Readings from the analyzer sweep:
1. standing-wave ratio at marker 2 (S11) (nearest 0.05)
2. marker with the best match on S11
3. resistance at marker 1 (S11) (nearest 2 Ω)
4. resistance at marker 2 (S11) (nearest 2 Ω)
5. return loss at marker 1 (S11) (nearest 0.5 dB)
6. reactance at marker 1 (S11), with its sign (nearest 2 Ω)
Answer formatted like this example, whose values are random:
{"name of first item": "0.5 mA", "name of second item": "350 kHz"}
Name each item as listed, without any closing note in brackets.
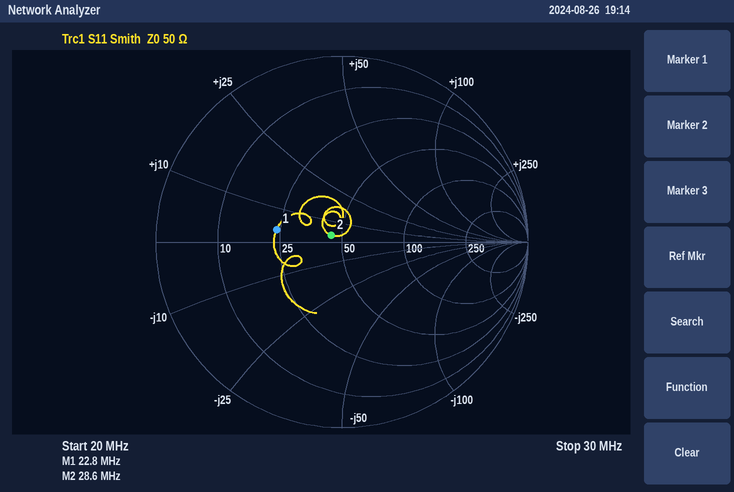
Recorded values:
{"standing-wave ratio at marker 2 (S11)": "1.15", "marker with the best match on S11": "marker 2", "resistance at marker 1 (S11)": "24 Ω", "resistance at marker 2 (S11)": "44 Ω", "return loss at marker 1 (S11)": "9.0 dB", "reactance at marker 1 (S11), with its sign": "+4 Ω"}
